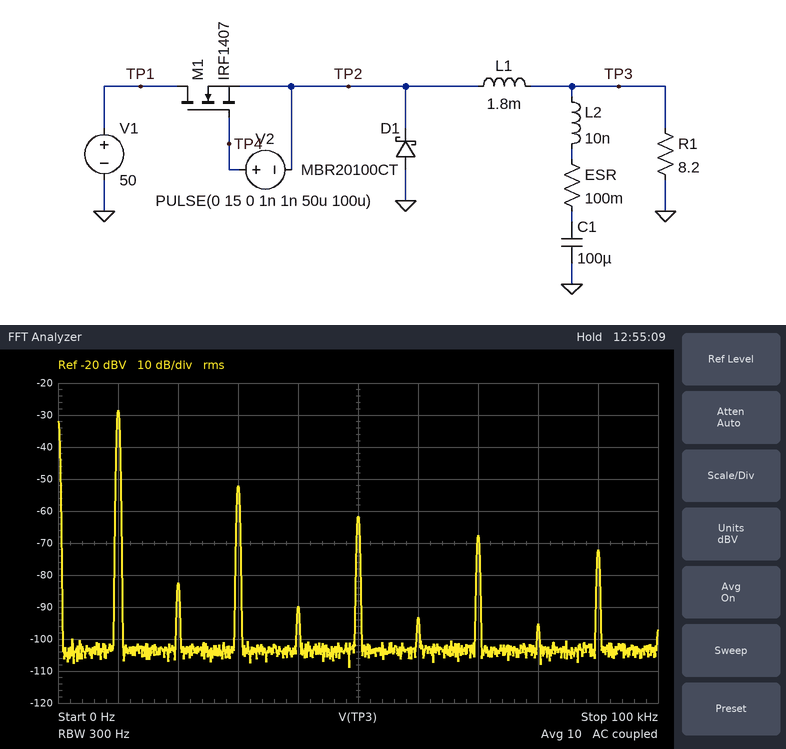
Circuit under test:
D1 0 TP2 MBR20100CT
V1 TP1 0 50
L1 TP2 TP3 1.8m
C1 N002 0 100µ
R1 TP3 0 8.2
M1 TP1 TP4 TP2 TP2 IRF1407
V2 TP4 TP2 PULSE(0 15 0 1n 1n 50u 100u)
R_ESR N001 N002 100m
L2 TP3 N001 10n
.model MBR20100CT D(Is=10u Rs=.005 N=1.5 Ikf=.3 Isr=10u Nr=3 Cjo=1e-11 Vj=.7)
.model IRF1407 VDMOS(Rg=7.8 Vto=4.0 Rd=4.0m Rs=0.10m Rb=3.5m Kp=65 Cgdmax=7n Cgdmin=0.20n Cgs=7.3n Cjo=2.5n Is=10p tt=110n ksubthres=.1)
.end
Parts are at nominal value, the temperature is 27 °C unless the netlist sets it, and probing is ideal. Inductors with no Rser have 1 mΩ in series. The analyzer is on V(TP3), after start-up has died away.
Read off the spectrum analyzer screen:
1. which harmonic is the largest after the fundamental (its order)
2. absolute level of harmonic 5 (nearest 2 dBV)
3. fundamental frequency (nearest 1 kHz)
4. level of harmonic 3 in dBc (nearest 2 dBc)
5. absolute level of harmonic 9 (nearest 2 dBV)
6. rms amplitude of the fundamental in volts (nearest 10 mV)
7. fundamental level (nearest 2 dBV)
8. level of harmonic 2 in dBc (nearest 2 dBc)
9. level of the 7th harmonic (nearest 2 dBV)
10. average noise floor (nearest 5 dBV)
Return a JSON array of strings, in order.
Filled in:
["3", "-62 dBV", "10 kHz", "-24 dBc", "-72 dBV", "40 mV", "-28 dBV", "-54 dBc", "-68 dBV", "-105 dBV"]
